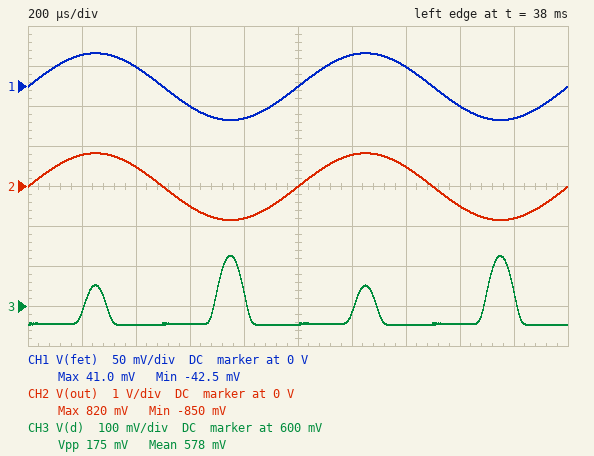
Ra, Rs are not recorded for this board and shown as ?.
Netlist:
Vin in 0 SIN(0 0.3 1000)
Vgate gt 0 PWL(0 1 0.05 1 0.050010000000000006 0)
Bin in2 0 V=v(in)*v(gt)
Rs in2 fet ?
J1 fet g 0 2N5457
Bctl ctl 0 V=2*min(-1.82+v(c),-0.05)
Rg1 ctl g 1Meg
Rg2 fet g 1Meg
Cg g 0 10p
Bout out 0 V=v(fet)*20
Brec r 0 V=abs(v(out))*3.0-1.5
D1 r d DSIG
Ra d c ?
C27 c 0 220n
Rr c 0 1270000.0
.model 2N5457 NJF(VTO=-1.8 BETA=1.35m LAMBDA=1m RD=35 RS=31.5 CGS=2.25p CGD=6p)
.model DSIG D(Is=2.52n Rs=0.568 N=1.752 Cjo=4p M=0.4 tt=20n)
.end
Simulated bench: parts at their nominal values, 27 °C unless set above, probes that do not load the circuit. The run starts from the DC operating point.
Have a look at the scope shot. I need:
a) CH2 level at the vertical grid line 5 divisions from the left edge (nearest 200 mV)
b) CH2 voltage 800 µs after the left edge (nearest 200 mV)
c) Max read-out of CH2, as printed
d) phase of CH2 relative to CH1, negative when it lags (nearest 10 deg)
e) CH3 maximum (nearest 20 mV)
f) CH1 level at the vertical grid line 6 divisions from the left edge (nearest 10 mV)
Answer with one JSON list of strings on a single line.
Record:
["0 V", "-800 mV", "820 mV", "0 deg", "720 mV", "40 mV"]
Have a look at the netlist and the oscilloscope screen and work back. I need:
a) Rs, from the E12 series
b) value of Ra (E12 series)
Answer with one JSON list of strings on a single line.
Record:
["4.7 kΩ", "47 kΩ"]
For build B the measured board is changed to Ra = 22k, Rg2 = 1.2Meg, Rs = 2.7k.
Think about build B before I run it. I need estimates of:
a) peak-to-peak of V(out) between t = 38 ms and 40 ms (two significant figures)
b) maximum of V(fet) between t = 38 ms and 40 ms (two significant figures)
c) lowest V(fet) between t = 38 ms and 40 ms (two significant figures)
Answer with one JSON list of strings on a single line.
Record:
["1.9 V", "48 mV", "-48 mV"]
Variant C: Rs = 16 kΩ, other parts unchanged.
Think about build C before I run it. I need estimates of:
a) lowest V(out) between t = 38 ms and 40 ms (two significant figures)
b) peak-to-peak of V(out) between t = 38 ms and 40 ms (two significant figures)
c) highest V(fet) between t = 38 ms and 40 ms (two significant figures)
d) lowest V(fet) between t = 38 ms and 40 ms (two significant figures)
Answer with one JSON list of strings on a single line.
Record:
["-710 mV", "1.3 V", "30 mV", "-35 mV"]
